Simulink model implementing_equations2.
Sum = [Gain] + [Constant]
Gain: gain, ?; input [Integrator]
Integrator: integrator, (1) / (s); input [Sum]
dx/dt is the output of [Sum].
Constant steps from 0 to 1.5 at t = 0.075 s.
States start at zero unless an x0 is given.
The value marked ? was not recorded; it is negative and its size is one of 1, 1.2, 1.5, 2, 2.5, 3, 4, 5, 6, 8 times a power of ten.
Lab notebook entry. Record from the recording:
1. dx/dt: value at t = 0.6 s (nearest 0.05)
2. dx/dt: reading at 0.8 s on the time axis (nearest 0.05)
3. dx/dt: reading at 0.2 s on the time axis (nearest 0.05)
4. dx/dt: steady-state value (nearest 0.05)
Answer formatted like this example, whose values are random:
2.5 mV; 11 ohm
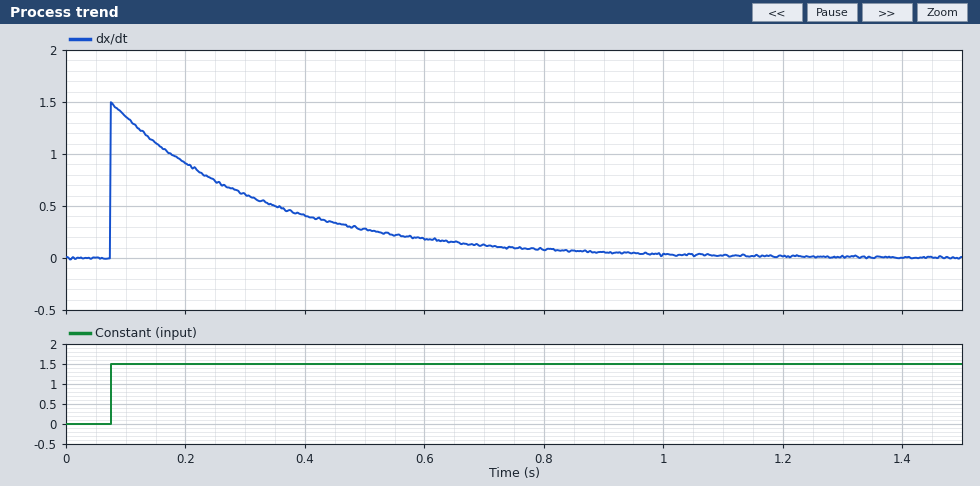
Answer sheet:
0.20; 0.10; 0.90; 0.00
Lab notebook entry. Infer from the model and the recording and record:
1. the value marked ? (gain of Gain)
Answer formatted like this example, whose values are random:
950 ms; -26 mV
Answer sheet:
-4
